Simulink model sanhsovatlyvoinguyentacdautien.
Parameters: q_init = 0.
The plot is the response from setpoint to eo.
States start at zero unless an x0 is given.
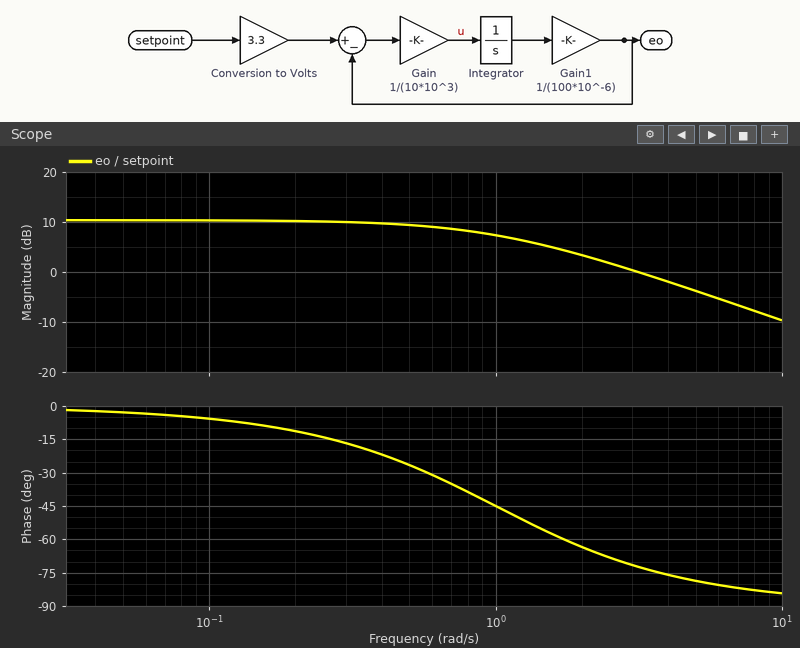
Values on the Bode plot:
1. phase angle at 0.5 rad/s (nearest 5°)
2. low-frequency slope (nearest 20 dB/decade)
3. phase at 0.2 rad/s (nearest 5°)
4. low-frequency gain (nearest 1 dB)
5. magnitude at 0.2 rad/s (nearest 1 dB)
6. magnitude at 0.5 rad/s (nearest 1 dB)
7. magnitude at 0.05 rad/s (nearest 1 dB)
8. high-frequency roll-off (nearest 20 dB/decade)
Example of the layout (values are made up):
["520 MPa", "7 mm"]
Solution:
["-25°", "0 dB/decade", "-10°", "10 dB", "10 dB", "9 dB", "10 dB", "-20 dB/decade"]
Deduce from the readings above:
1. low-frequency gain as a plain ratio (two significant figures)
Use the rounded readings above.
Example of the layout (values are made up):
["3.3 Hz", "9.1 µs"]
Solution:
["3.2"]
